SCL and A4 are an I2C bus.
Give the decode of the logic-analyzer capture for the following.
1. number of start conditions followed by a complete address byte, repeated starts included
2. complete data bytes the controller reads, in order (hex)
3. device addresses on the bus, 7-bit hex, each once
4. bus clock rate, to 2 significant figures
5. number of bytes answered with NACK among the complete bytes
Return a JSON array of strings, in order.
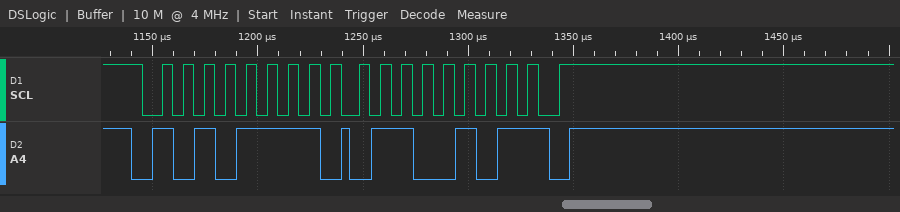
["1", "65", "0x57", "100 kHz", "1"]
